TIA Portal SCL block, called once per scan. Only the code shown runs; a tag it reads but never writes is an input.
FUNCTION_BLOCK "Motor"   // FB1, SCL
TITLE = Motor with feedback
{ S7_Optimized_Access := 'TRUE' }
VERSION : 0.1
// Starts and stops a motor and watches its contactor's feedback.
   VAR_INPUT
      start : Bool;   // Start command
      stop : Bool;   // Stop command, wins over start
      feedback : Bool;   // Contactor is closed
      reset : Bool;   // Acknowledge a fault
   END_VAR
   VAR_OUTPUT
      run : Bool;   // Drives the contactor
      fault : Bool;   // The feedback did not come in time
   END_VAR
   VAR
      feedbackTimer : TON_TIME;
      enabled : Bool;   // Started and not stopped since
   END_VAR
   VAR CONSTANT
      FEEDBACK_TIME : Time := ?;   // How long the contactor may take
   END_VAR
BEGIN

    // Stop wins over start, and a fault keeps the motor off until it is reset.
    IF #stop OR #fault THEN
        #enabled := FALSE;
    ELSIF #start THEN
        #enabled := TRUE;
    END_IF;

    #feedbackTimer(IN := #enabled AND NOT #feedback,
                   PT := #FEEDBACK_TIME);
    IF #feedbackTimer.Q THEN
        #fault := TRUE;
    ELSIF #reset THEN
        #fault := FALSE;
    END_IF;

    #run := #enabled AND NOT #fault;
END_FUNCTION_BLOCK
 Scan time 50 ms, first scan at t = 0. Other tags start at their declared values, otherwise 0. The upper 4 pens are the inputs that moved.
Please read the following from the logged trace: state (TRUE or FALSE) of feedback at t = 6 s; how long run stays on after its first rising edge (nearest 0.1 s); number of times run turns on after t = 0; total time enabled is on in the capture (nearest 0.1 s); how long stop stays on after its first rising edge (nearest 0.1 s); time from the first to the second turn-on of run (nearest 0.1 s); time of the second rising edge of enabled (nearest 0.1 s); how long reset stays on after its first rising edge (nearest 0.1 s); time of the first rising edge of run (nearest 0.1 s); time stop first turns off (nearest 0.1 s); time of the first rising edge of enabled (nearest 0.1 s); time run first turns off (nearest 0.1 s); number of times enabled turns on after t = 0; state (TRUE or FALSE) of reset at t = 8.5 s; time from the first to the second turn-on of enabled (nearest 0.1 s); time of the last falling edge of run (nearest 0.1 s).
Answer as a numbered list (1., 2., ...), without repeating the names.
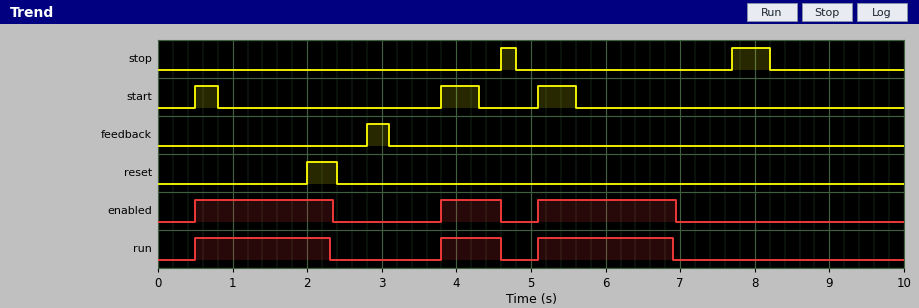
1. FALSE
2. 1.8 s
3. 3
4. 4.5 s
5. 0.2 s
6. 3.3 s
7. 3.8 s
8. 0.4 s
9. 0.5 s
10. 4.8 s
11. 0.5 s
12. 2.3 s
13. 3
14. FALSE
15. 3.3 s
16. 6.9 s
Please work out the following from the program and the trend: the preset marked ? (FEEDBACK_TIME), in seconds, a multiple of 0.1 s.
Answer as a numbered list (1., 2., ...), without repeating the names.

1. 1.8 s
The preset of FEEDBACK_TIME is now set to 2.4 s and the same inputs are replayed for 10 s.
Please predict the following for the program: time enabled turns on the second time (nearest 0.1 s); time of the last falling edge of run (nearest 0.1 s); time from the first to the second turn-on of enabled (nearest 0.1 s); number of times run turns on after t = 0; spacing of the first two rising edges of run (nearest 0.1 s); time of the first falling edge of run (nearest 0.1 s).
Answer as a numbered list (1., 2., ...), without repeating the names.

1. 5.1 s
2. 7.5 s
3. 4.6 s
4. 2
5. 4.6 s
6. 4.6 s
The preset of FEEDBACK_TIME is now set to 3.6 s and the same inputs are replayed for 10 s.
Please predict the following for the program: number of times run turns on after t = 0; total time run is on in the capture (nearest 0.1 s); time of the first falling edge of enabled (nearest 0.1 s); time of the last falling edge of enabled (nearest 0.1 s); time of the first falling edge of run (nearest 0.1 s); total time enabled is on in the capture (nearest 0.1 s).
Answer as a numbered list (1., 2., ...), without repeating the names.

1. 2
2. 6.7 s
3. 4.6 s
4. 7.7 s
5. 4.6 s
6. 6.7 s
